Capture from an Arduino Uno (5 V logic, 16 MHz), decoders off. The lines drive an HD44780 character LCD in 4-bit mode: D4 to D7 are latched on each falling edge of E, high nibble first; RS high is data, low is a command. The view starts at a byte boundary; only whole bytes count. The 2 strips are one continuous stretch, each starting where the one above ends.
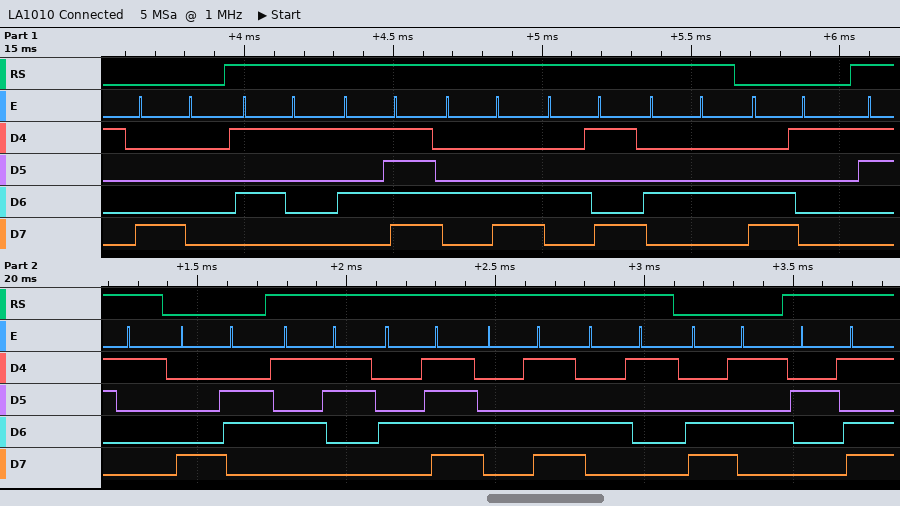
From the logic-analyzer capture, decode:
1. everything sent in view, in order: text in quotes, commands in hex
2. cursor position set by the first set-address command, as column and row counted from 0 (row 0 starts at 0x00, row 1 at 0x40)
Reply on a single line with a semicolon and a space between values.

0x80 "Q_LID" 0xC1 "1" 0x86 "SOMA" 0xC5 "-"; column 0, row 0
